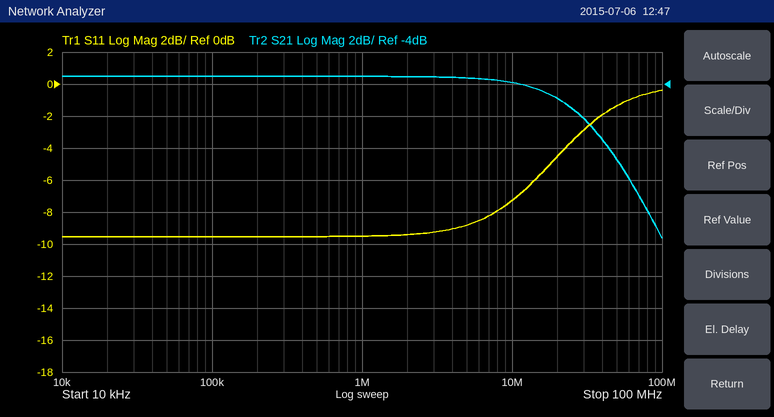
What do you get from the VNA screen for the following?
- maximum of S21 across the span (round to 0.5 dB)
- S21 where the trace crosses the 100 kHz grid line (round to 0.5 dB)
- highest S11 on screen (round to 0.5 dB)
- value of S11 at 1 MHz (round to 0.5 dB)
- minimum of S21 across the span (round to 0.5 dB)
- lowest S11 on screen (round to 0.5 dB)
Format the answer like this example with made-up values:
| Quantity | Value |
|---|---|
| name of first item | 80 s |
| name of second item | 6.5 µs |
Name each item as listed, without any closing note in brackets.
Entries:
| Quantity | Value |
|---|---|
| maximum of S21 across the span | -3.5 dB |
| S21 where the trace crosses the 100 kHz grid line | -3.5 dB |
| highest S11 on screen | -0.5 dB |
| value of S11 at 1 MHz | -9.5 dB |
| minimum of S21 across the span | -13.5 dB |
| lowest S11 on screen | -9.5 dB |
